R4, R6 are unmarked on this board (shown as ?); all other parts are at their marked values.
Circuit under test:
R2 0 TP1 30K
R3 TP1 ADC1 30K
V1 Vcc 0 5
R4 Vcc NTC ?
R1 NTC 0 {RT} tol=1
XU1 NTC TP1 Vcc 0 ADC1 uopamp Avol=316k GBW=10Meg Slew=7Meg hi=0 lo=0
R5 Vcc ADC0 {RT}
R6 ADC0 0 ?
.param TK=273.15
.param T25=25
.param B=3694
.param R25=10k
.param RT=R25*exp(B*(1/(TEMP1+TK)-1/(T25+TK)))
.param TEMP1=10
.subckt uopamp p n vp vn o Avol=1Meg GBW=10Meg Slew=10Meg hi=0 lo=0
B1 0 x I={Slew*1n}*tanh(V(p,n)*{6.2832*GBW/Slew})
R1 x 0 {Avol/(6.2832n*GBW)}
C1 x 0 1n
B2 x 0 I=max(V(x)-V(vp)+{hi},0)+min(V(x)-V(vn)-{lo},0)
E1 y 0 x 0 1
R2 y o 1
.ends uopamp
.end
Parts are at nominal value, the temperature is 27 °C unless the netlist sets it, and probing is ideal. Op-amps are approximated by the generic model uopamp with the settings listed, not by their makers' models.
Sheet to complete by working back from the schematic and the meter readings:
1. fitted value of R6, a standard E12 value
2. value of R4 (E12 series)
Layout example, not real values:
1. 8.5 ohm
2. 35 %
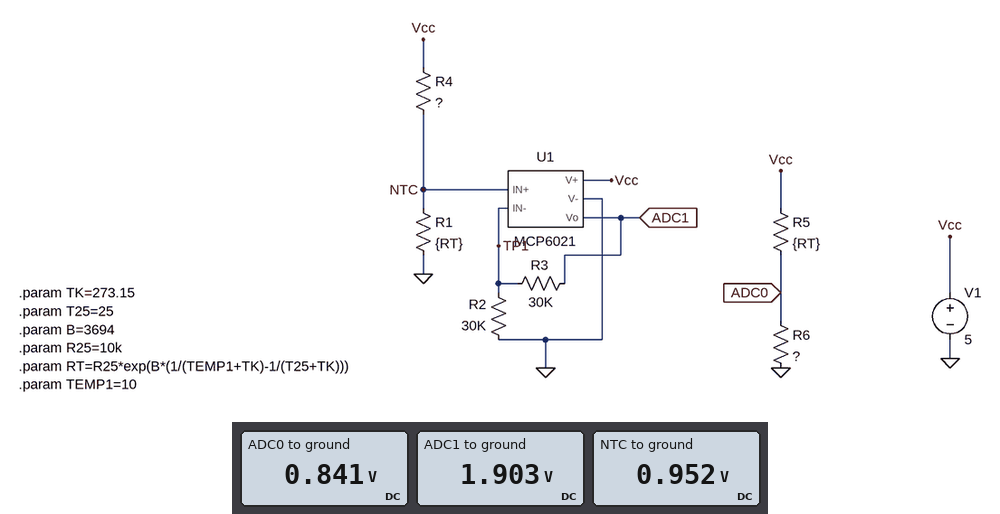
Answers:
1. 3.9 kΩ
2. 82 kΩ
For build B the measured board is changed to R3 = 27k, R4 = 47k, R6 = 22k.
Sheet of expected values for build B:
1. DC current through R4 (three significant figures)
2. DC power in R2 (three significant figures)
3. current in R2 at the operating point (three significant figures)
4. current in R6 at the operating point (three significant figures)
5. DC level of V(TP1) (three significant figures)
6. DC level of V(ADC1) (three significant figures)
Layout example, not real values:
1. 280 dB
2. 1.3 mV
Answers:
1. 75.4 µA
2. 70.5 µW
3. 48.5 µA
4. 121 µA
5. 1.45 V
6. 2.76 V
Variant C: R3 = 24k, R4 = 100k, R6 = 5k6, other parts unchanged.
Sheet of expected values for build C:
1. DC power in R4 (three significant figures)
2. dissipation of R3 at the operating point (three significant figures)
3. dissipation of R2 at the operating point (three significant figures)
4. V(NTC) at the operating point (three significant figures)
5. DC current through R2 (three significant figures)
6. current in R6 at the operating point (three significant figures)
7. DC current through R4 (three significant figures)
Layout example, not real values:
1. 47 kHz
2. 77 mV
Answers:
1. 176 µW
2. 17.4 µW
3. 21.8 µW
4. 808 mV
5. 26.9 µA
6. 201 µA
7. 41.9 µA
